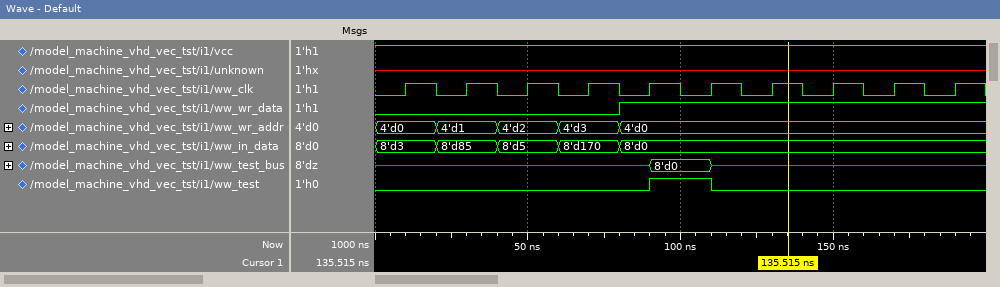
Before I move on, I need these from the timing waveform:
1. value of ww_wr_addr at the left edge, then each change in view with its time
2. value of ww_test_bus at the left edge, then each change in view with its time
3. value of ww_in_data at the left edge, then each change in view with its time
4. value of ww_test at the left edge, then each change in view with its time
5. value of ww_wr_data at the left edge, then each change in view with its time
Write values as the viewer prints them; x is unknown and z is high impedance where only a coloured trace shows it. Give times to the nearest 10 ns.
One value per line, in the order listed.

4'd0, 4'd1 at 20 ns, 4'd2 at 40 ns, 4'd3 at 60 ns, 4'd0 at 80 ns
z, 8'd0 at 90 ns, z at 110 ns
8'd3, 8'd85 at 20 ns, 8'd5 at 40 ns, 8'd170 at 60 ns, 8'd0 at 80 ns
0, 1 at 90 ns, 0 at 110 ns
0, 1 at 80 ns
